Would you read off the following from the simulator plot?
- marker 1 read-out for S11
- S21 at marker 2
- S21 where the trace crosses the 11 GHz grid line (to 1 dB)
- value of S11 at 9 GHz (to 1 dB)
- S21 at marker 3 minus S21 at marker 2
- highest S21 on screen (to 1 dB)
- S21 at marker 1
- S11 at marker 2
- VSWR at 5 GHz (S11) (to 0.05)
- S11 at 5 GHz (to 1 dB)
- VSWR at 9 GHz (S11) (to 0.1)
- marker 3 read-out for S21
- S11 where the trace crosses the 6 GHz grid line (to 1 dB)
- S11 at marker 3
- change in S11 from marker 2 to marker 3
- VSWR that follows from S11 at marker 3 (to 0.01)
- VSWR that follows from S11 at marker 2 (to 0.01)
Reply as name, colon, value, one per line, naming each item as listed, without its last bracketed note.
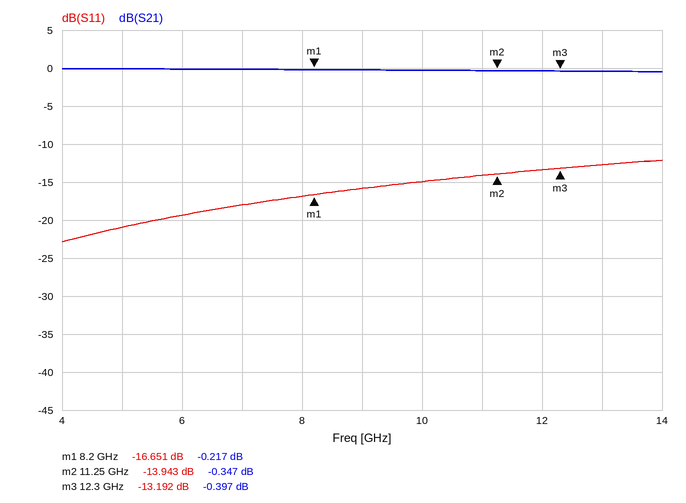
marker 1 read-out for S11: -16.651 dB
S21 at marker 2: -0.347 dB
S21 where the trace crosses the 11 GHz grid line: 0 dB
value of S11 at 9 GHz: -16 dB
S21 at marker 3 minus S21 at marker 2: -0.050 dB
highest S21 on screen: 0 dB
S21 at marker 1: -0.217 dB
S11 at marker 2: -13.943 dB
VSWR at 5 GHz (S11): 1.20
S11 at 5 GHz: -21 dB
VSWR at 9 GHz (S11): 1.4
marker 3 read-out for S21: -0.397 dB
S11 where the trace crosses the 6 GHz grid line: -19 dB
S11 at marker 3: -13.192 dB
change in S11 from marker 2 to marker 3: 0.751 dB
VSWR that follows from S11 at marker 3: 1.56
VSWR that follows from S11 at marker 2: 1.50
